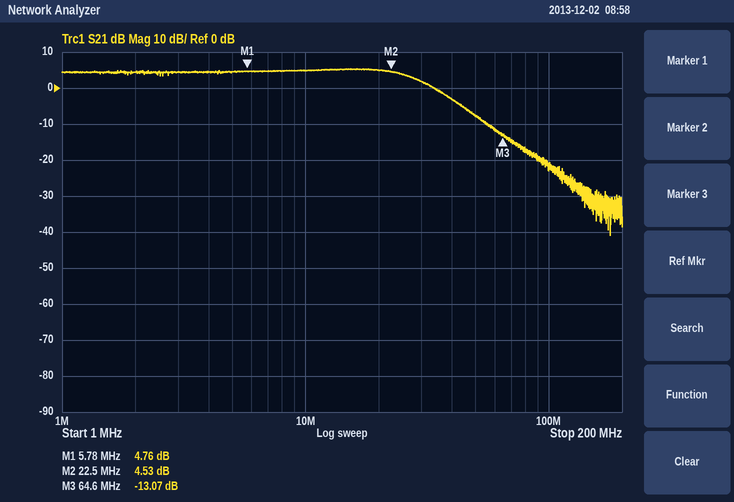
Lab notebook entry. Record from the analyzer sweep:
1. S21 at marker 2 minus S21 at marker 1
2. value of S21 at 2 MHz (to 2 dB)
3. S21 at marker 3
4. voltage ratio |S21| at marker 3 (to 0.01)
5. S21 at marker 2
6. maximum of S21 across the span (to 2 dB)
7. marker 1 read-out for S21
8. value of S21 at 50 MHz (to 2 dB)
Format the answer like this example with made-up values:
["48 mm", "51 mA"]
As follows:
["-0.23 dB", "4 dB", "-13.07 dB", "0.22", "4.53 dB", "6 dB", "4.76 dB", "-8 dB"]
